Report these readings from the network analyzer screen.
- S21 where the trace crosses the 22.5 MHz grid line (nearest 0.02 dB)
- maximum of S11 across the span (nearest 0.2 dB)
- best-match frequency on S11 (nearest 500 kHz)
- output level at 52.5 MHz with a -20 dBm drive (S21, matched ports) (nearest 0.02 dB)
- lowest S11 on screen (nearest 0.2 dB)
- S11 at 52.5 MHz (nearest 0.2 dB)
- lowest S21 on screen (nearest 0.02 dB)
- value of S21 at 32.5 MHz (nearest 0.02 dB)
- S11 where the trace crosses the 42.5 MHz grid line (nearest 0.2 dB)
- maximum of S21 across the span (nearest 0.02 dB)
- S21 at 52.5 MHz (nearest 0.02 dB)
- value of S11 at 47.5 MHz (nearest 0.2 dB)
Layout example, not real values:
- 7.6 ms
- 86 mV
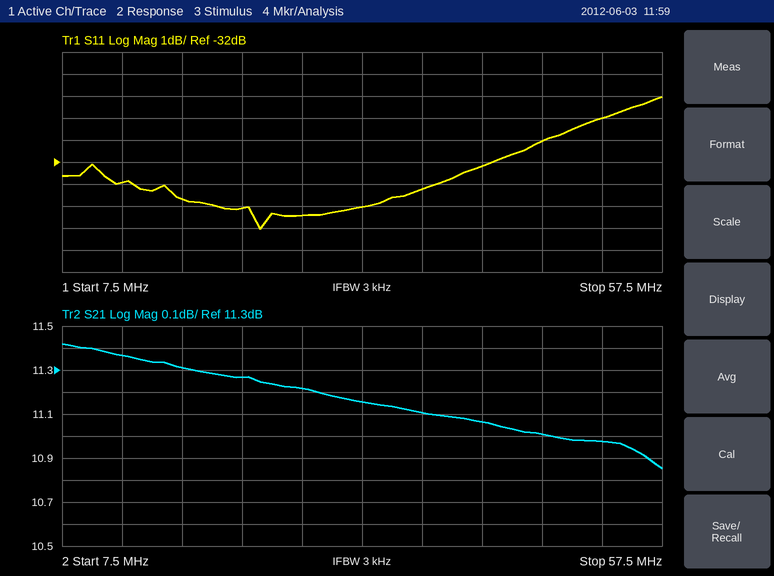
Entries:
- 11.26 dB
- -29.0 dB
- 24.0 MHz
- -9.02 dBm
- -35.0 dB
- -30.0 dB
- 10.86 dB
- 11.16 dB
- -32.2 dB
- 11.42 dB
- 10.98 dB
- -31.0 dB
